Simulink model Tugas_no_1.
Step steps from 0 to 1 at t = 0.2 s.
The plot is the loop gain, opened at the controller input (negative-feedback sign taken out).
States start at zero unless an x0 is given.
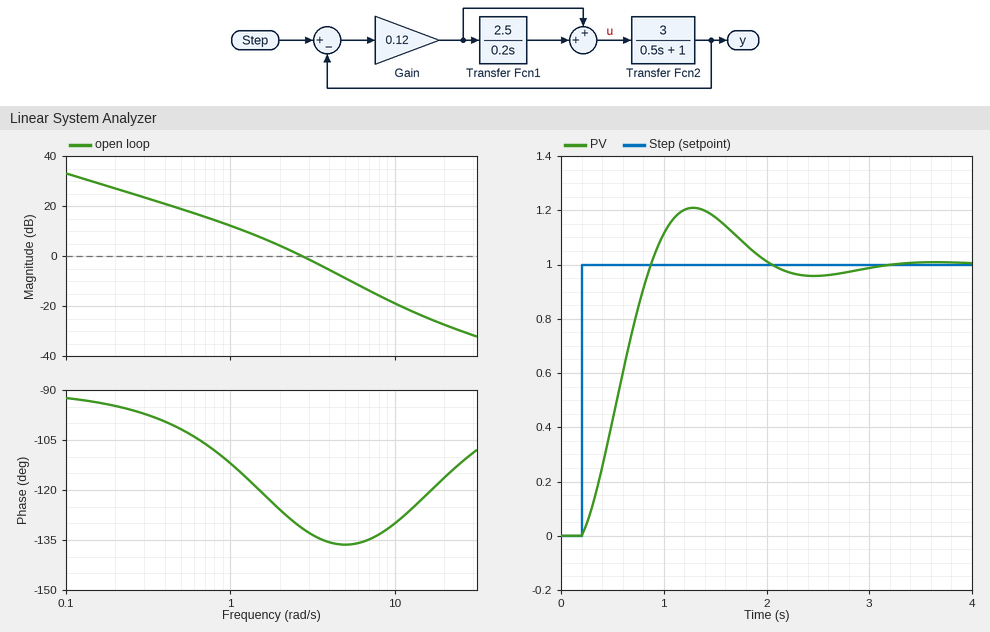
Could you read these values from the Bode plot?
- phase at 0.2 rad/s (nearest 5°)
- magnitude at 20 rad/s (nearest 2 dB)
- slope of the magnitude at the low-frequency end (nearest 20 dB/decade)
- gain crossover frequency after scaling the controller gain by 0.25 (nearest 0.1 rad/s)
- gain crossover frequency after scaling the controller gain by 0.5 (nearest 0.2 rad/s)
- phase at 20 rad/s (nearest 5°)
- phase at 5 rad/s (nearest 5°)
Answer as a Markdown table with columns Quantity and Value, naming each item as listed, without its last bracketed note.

| Quantity | Value |
|---|---|
| phase at 0.2 rad/s | -95° |
| magnitude at 20 rad/s | -28 dB |
| slope of the magnitude at the low-frequency end | -20 dB/decade |
| gain crossover frequency after scaling the controller gain by 0.25 | 1.0 rad/s |
| gain crossover frequency after scaling the controller gain by 0.5 | 1.8 rad/s |
| phase at 20 rad/s | -115° |
| phase at 5 rad/s | -135° |
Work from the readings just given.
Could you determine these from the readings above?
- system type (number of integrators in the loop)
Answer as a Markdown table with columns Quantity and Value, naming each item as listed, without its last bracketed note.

| Quantity | Value |
|---|---|
| system type | 1 |
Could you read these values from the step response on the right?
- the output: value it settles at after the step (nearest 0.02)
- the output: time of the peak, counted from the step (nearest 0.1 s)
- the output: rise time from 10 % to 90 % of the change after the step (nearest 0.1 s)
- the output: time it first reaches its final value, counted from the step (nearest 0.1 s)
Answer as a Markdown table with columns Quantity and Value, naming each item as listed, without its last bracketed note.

| Quantity | Value |
|---|---|
| the output: value it settles at after the step | 1.00 |
| the output: time of the peak, counted from the step | 1.1 s |
| the output: rise time from 10 % to 90 % of the change after the step | 0.5 s |
| the output: time it first reaches its final value, counted from the step | 0.7 s |
